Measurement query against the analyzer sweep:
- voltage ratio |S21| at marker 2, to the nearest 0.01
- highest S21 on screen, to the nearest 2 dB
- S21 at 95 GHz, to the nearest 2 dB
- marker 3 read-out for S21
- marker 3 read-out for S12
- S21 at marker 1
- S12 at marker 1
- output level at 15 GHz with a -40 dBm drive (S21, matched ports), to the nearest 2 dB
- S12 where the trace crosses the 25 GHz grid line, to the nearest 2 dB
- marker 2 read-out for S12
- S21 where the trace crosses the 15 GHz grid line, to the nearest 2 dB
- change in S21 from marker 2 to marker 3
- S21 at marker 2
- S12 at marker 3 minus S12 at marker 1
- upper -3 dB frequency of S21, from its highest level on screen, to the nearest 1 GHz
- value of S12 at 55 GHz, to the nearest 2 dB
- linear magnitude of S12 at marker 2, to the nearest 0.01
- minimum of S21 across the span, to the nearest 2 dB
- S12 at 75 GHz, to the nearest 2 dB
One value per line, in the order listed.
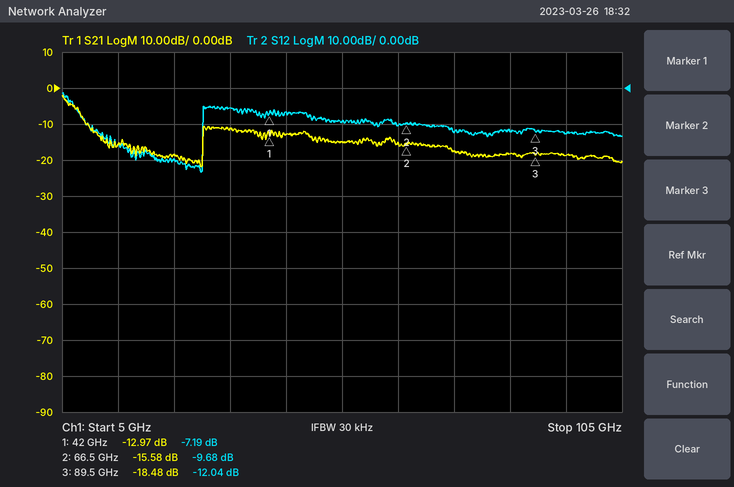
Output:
0.17
-2 dB
-18 dB
-18.48 dB
-12.04 dB
-12.97 dB
-7.19 dB
-56 dBm
-20 dB
-9.68 dB
-16 dB
-2.90 dB
-15.58 dB
-4.85 dB
7 GHz
-10 dB
0.33
-22 dB
-12 dB
